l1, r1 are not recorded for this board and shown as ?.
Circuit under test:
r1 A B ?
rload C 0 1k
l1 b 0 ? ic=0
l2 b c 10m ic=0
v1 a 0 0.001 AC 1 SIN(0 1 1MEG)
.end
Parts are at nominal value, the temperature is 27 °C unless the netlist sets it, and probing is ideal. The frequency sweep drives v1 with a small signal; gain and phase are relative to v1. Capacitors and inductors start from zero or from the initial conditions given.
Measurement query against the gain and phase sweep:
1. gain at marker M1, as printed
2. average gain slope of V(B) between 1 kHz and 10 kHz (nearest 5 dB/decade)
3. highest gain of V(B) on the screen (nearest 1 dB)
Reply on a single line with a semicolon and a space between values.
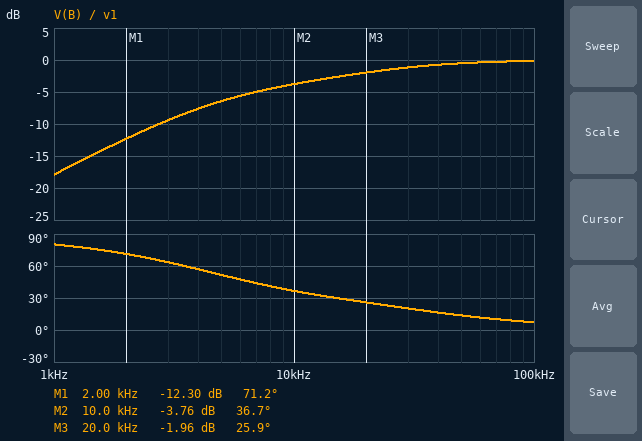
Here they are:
-12.30 dB; 15 dB/decade; 0 dB
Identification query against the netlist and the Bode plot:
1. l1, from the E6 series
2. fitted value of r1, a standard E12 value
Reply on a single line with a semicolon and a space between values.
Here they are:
6.8 mH; 330 Ω
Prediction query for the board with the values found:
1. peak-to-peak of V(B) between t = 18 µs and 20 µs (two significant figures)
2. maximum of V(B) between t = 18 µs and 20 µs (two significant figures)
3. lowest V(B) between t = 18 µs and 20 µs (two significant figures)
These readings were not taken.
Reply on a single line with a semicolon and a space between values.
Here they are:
2.0 V; 1.0 V; -1.0 V
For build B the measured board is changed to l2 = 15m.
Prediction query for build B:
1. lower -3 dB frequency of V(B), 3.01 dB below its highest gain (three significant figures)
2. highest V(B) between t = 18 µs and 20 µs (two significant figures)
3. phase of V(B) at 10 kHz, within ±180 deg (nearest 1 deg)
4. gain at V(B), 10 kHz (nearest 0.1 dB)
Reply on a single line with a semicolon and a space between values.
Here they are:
11.7 kHz; 1.0 V; 39 deg; -3.5 dB
